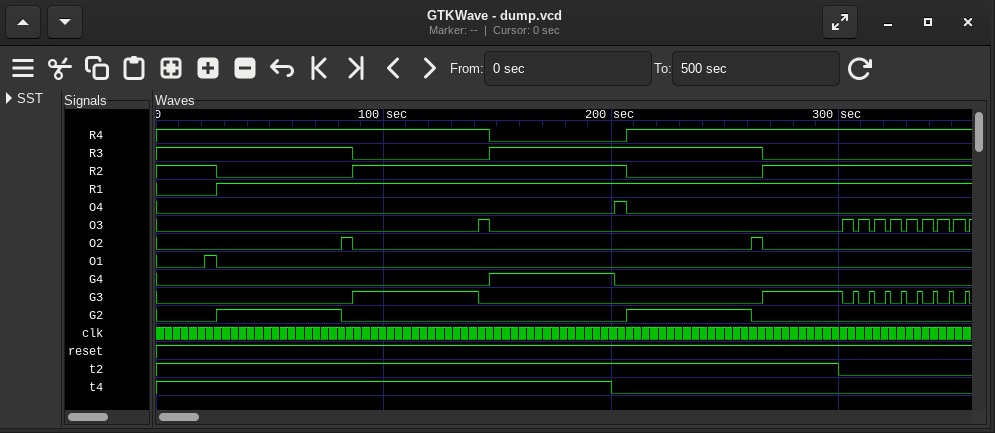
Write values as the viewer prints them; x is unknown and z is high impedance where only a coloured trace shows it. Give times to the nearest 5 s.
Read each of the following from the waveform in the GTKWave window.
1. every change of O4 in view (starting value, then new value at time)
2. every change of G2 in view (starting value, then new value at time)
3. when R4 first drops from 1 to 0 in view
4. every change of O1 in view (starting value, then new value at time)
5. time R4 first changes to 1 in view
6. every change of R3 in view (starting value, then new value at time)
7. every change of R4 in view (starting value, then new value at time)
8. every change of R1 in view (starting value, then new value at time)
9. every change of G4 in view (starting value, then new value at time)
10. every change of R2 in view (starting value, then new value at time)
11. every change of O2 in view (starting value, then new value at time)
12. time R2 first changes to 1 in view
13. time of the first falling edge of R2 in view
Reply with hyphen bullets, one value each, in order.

- 0, 1 at 200 s, 0 at 205 s
- 0, 1 at 25 s, 0 at 80 s, 1 at 205 s, 0 at 260 s
- 145 s
- 0, 1 at 20 s, 0 at 25 s
- 205 s
- 1, 0 at 85 s, 1 at 145 s, 0 at 265 s
- 1, 0 at 145 s, 1 at 205 s
- 0, 1 at 25 s
- 0, 1 at 145 s, 0 at 200 s
- 1, 0 at 25 s, 1 at 85 s, 0 at 205 s, 1 at 265 s
- 0, 1 at 80 s, 0 at 85 s, 1 at 260 s, 0 at 265 s
- 85 s
- 25 s
